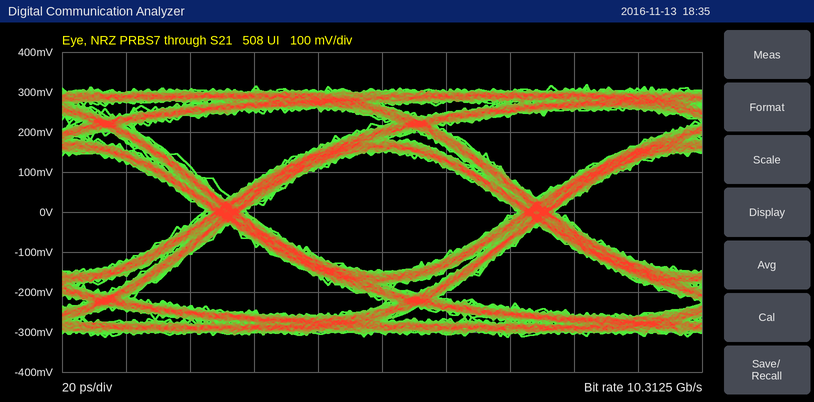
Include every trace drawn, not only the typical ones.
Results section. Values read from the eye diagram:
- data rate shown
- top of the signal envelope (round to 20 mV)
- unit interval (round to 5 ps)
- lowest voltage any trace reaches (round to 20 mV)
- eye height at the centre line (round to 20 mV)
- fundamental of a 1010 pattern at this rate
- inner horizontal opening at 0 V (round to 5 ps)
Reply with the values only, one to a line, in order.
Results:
10.3125 Gb/s
320 mV
95 ps
-320 mV
300 mV
5.15625 GHz
85 ps
